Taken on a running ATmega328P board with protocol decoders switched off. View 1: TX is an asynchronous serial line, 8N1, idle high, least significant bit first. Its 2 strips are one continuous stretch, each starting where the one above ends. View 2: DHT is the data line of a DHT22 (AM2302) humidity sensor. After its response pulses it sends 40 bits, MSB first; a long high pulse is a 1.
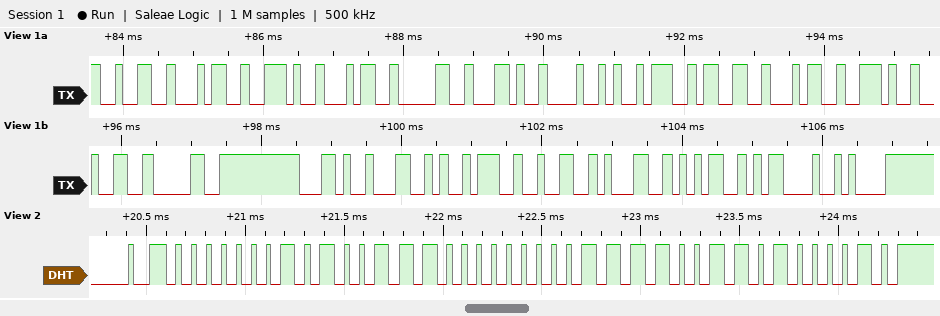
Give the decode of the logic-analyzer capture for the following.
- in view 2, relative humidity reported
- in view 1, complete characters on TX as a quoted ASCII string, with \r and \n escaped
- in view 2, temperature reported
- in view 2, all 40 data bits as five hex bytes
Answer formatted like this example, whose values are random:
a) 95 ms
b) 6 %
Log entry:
a) 33.4 %
b) "24.40,H:34.20,L:215\r\n"
c) 24.3 °C
d) 01 4E 00 F3 42
